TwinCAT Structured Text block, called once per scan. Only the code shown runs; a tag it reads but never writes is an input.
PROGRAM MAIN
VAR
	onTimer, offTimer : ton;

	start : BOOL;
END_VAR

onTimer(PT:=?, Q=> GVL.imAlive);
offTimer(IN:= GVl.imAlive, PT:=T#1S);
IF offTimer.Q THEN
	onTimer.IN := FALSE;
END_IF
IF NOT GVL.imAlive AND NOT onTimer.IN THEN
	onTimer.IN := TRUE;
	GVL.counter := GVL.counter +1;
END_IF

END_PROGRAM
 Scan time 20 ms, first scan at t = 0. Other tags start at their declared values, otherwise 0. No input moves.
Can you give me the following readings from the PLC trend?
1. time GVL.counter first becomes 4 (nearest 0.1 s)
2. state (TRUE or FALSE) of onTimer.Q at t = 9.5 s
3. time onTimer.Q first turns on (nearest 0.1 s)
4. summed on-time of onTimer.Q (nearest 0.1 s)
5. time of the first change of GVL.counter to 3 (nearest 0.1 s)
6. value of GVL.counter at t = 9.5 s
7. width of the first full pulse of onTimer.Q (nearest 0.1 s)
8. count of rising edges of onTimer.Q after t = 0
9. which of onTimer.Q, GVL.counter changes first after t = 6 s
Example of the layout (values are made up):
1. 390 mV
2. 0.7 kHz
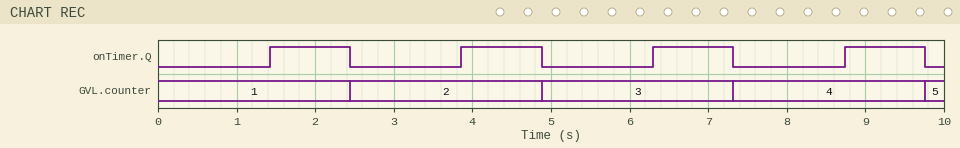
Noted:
1. 7.3 s
2. TRUE
3. 1.4 s
4. 4.1 s
5. 4.9 s
6. 4
7. 1.0 s
8. 4
9. onTimer.Q
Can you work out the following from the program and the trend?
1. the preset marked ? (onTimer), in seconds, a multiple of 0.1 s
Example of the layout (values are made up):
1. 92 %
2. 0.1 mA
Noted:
1. 1.4 s
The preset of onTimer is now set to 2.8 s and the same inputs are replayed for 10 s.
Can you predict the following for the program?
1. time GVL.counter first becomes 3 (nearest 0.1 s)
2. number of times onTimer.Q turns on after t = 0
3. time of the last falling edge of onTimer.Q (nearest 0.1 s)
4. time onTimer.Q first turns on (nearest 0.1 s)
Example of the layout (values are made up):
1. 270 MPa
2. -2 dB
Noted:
1. 7.7 s
2. 2
3. 7.7 s
4. 2.8 s
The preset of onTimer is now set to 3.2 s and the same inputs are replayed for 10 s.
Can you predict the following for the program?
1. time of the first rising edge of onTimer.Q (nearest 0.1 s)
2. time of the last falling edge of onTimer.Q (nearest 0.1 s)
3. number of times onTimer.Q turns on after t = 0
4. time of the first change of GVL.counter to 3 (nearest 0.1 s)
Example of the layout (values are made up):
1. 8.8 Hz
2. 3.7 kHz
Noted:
1. 3.2 s
2. 8.5 s
3. 2
4. 8.5 s
